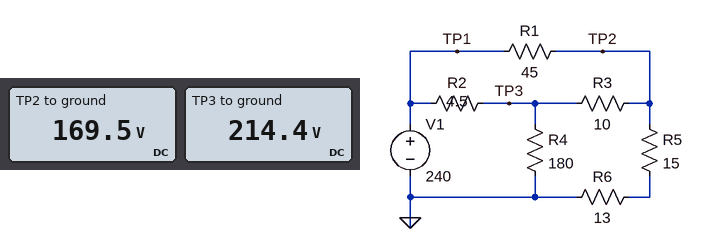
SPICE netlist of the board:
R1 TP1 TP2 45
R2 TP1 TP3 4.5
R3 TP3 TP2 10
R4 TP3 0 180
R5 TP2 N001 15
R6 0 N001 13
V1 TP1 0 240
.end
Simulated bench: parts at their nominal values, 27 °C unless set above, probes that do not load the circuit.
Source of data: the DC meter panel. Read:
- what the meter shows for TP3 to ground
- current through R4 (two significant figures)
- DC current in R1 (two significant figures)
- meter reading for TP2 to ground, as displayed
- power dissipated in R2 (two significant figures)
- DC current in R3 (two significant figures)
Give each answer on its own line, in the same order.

214.4 V
1.2 A
1.6 A
169.5 V
150 W
4.5 A
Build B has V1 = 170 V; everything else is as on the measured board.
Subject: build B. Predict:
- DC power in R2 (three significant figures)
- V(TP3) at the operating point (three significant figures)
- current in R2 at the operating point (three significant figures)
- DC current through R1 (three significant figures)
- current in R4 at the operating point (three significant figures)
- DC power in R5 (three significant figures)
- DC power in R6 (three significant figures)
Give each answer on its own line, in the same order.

72.9 W
152 V
4.02 A
1.11 A
844 mA
276 W
239 W
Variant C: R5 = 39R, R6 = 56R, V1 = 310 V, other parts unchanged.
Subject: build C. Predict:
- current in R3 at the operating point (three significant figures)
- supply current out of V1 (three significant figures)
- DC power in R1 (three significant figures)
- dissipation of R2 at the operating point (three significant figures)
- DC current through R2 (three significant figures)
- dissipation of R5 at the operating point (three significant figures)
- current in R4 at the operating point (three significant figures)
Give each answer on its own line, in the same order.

2.05 A
4.50 A
30.5 W
60.9 W
3.68 A
322 W
1.63 A
